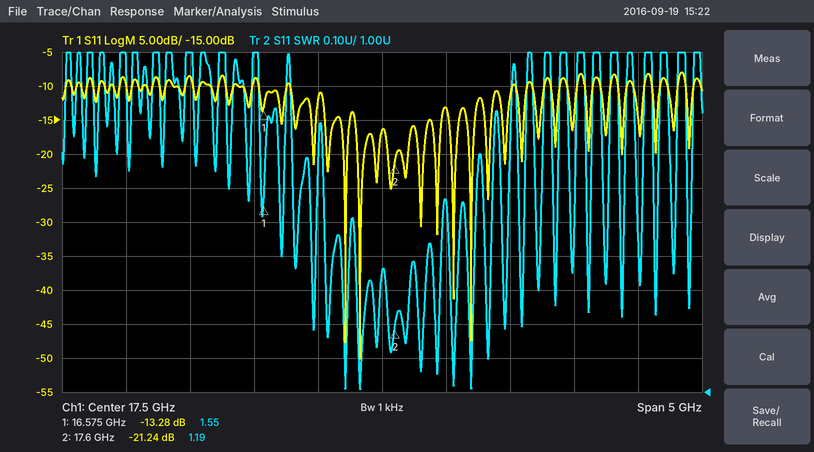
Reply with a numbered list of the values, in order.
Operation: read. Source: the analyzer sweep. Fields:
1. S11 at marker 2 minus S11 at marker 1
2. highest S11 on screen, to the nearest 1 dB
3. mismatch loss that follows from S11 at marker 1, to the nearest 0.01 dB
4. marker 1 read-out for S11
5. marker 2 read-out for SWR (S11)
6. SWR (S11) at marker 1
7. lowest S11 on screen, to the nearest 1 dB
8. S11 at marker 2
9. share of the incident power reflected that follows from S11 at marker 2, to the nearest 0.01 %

1. -7.96 dB
2. -8 dB
3. 0.21 dB
4. -13.28 dB
5. 1.19
6. 1.55
7. -50 dB
8. -21.24 dB
9. 0.75 %
